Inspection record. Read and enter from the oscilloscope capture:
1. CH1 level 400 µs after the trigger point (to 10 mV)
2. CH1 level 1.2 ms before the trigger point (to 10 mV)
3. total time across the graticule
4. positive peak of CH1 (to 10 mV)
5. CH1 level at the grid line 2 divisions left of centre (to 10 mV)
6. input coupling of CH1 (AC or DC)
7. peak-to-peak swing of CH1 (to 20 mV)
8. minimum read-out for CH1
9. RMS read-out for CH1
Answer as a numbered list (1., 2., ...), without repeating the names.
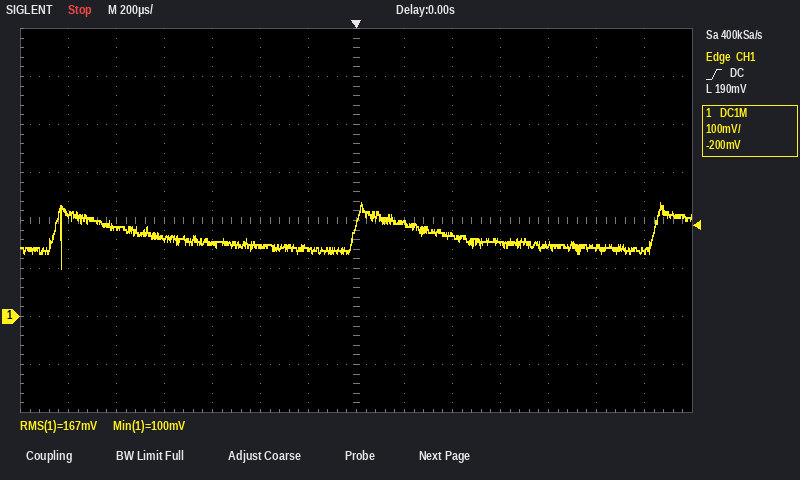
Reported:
1. 170 mV
2. 210 mV
3. 2.8 ms
4. 240 mV
5. 150 mV
6. DC
7. 140 mV
8. 100 mV
9. 167 mV
